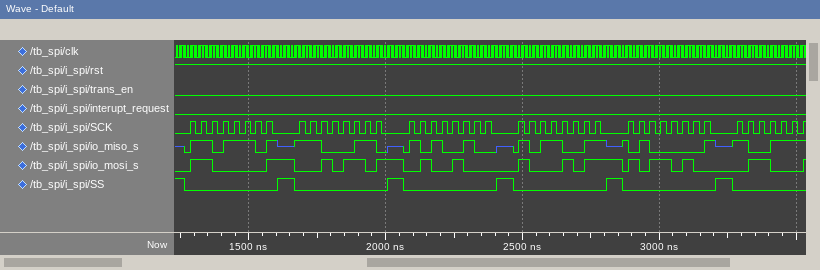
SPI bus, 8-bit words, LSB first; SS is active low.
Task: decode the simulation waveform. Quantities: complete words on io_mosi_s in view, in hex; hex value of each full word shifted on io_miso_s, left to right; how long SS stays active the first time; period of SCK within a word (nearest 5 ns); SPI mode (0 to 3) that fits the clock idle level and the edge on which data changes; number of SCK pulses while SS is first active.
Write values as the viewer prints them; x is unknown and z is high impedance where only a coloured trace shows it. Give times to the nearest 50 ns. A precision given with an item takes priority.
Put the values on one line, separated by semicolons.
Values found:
83, B4, 12, D1, 2D; BB, 63, 25, CD, 82; 350 ns; 40 ns; 1; 8
